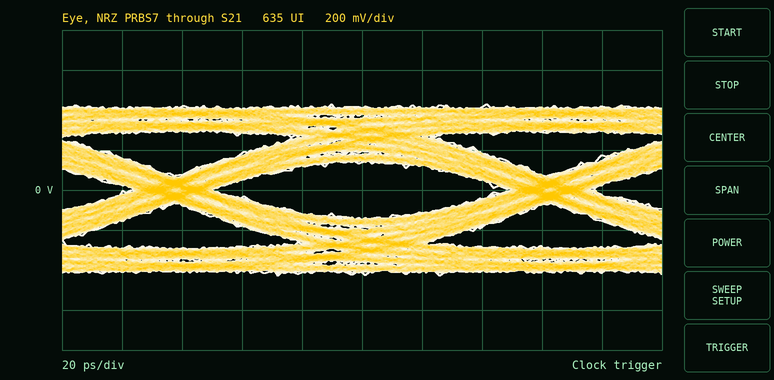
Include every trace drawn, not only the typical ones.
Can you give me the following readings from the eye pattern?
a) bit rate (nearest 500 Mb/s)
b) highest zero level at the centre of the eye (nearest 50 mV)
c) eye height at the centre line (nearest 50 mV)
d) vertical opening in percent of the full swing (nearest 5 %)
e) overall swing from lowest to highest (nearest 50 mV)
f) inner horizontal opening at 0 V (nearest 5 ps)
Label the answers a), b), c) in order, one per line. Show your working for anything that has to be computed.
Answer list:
a) 8.0 Gb/s
b) -150 mV
c) 300 mV
d) 300 mV / 850 mV ≈ 35 %
e) 850 mV
f) 100 ps
